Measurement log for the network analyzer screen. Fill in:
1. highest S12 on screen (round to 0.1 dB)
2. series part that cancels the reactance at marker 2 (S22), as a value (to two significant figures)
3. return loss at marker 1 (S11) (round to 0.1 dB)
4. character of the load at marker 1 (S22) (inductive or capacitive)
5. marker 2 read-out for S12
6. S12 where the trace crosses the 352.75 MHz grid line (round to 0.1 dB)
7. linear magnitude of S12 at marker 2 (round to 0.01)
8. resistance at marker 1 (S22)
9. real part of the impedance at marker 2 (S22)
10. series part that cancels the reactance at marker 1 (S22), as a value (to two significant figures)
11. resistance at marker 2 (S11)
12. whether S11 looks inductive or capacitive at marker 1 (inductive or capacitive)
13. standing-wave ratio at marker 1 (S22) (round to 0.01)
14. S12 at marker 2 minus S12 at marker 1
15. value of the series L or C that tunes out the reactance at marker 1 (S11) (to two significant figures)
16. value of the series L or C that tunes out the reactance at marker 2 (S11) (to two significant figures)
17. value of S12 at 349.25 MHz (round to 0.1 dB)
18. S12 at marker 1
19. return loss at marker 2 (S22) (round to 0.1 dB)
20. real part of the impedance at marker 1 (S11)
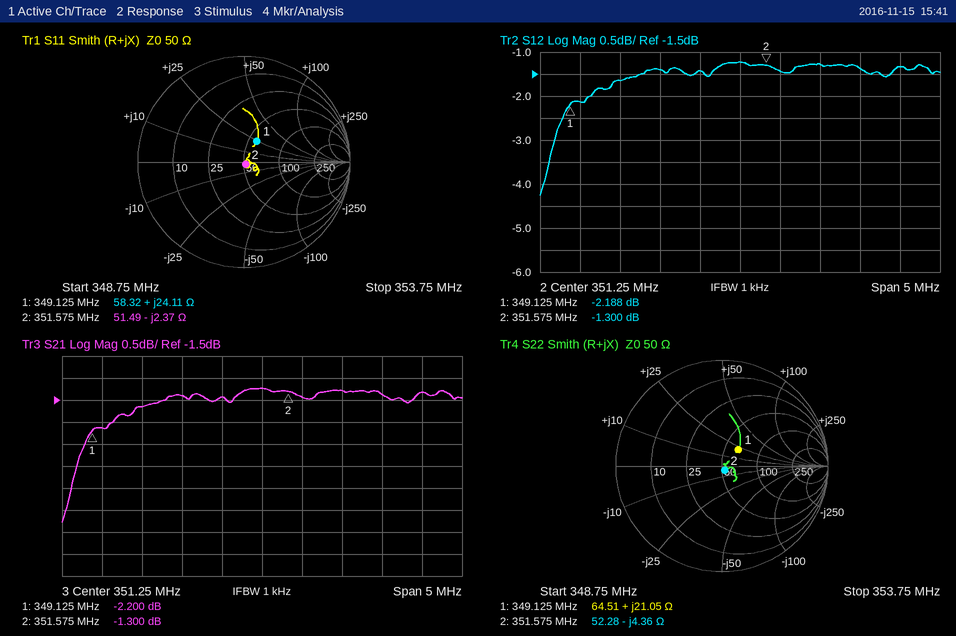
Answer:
-1.2 dB
2.0 nH
12.8 dB
inductive
-1.300 dB
-1.4 dB
0.86
64.51 Ω
52.28 Ω
22 pF
51.49 Ω
inductive
1.56
0.888 dB
19 pF
1.1 nH
-2.1 dB
-2.188 dB
26.4 dB
58.32 Ω
